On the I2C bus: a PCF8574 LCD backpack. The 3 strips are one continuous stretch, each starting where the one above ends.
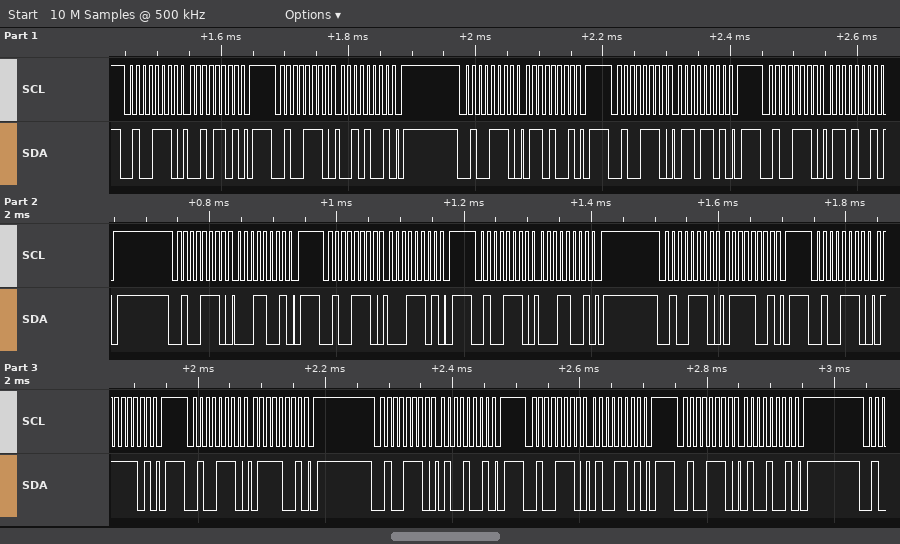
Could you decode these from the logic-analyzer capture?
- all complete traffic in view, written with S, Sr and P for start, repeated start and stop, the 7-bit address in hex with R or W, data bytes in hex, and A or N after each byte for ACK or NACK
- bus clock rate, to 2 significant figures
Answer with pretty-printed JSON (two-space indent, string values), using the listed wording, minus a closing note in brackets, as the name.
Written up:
{
  "all complete traffic in view, written with S, Sr and P for start, repeated start and stop, the 7-bit address in hex with R or W, data bytes in hex, and A or N after each byte for ACK or NACK": "S 27W A 2D A P S 27W A 29 A P S 27W A 69 A P S 27W A 6D A P S 27W A 69 A P S 27W A 19 A P S 27W A 1D A P S 27W A 19 A P S 27W A 79 A P S 27W A 7D A P S 27W A 79 A P S 27W A 49 A P S 27W A 4D A P S 27W A 49 A P",
  "bus clock rate, to 2 significant figures": "100 kHz"
}
